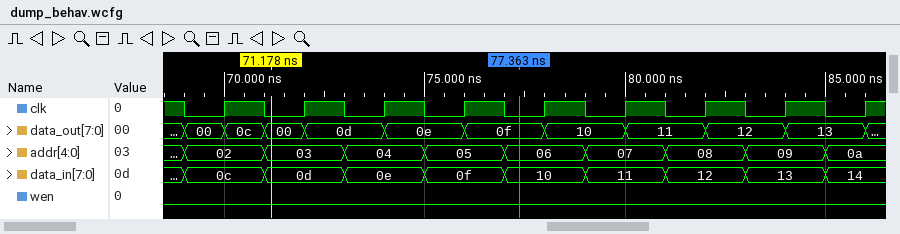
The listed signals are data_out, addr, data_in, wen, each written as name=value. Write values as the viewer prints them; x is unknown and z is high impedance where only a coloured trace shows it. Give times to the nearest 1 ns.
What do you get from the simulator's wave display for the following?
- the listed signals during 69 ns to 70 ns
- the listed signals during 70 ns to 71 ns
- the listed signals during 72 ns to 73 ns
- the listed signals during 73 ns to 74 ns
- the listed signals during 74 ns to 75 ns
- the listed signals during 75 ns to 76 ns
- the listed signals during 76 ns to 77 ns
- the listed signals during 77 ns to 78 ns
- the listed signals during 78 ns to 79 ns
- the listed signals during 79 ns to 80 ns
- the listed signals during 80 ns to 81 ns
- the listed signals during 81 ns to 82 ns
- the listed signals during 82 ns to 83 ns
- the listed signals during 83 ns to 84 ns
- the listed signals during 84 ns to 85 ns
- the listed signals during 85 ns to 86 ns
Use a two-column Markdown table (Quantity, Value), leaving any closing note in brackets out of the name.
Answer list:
| Quantity | Value |
|---|---|
| the listed signals during 69 ns to 70 ns | data_out=00, addr=02, data_in=0c, wen=0 |
| the listed signals during 70 ns to 71 ns | data_out=0c, addr=02, data_in=0c, wen=0 |
| the listed signals during 72 ns to 73 ns | data_out=0d, addr=03, data_in=0d, wen=0 |
| the listed signals during 73 ns to 74 ns | data_out=0d, addr=04, data_in=0e, wen=0 |
| the listed signals during 74 ns to 75 ns | data_out=0e, addr=04, data_in=0e, wen=0 |
| the listed signals during 75 ns to 76 ns | data_out=0e, addr=05, data_in=0f, wen=0 |
| the listed signals during 76 ns to 77 ns | data_out=0f, addr=05, data_in=0f, wen=0 |
| the listed signals during 77 ns to 78 ns | data_out=0f, addr=06, data_in=10, wen=0 |
| the listed signals during 78 ns to 79 ns | data_out=10, addr=06, data_in=10, wen=0 |
| the listed signals during 79 ns to 80 ns | data_out=10, addr=07, data_in=11, wen=0 |
| the listed signals during 80 ns to 81 ns | data_out=11, addr=07, data_in=11, wen=0 |
| the listed signals during 81 ns to 82 ns | data_out=11, addr=08, data_in=12, wen=0 |
| the listed signals during 82 ns to 83 ns | data_out=12, addr=08, data_in=12, wen=0 |
| the listed signals during 83 ns to 84 ns | data_out=12, addr=09, data_in=13, wen=0 |
| the listed signals during 84 ns to 85 ns | data_out=13, addr=09, data_in=13, wen=0 |
| the listed signals during 85 ns to 86 ns | data_out=13, addr=0a, data_in=14, wen=0 |
